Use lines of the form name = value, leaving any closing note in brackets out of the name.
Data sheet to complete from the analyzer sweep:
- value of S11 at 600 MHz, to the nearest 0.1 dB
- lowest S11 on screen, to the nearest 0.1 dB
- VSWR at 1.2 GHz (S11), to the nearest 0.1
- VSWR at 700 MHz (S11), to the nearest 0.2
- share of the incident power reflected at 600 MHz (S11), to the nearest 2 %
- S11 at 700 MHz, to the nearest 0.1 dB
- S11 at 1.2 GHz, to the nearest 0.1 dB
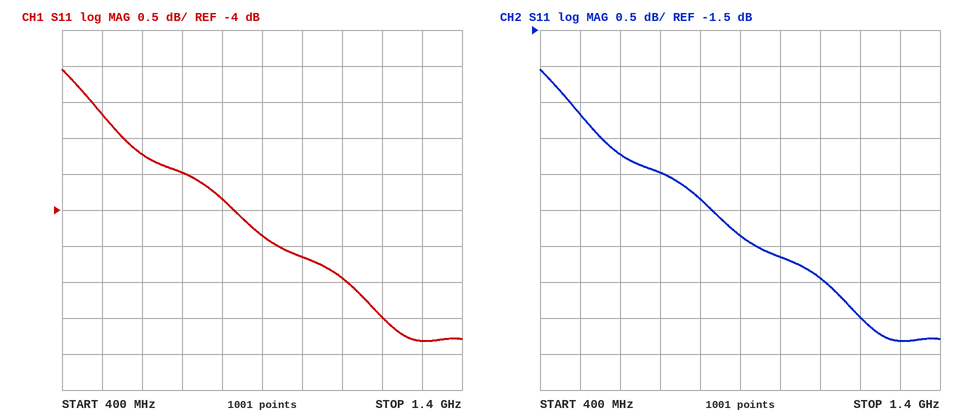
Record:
value of S11 at 600 MHz, to the nearest 0.1 dB = -3.2 dB
lowest S11 on screen, to the nearest 0.1 dB = -5.8 dB
VSWR at 1.2 GHz (S11), to the nearest 0.1 = 3.3
VSWR at 700 MHz (S11), to the nearest 0.2 = 5.0
share of the incident power reflected at 600 MHz (S11), to the nearest 2 % = 48 %
S11 at 700 MHz, to the nearest 0.1 dB = -3.5 dB
S11 at 1.2 GHz, to the nearest 0.1 dB = -5.5 dB
